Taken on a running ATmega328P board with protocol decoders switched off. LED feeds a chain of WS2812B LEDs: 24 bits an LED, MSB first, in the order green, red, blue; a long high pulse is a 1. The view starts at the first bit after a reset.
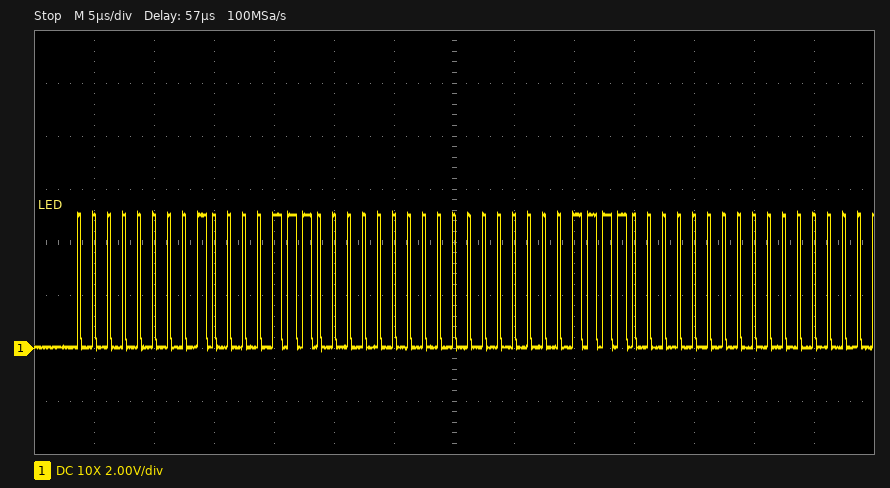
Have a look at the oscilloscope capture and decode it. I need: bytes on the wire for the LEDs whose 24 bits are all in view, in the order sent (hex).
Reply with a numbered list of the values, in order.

1. 00 87 00 00 78 00
